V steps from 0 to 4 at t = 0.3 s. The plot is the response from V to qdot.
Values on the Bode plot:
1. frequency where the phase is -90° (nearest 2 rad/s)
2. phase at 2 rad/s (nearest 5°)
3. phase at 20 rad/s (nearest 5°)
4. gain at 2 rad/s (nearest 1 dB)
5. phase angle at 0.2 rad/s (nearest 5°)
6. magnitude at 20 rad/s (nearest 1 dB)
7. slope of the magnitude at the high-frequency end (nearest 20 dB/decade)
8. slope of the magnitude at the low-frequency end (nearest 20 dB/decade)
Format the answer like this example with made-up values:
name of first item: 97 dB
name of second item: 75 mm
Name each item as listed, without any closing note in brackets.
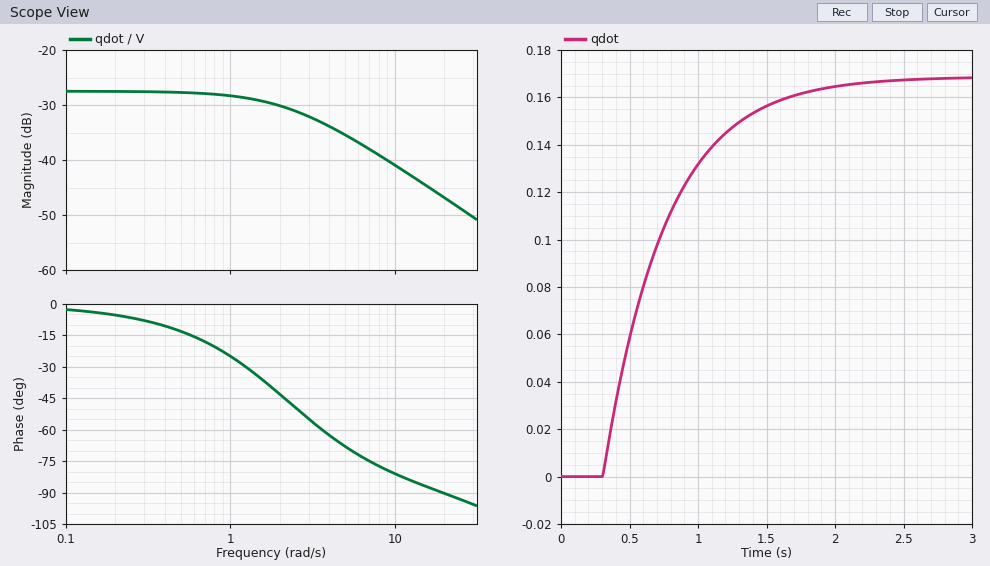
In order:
frequency where the phase is -90°: 20 rad/s
phase at 2 rad/s: -45°
phase at 20 rad/s: -90°
gain at 2 rad/s: -30 dB
phase angle at 0.2 rad/s: -5°
magnitude at 20 rad/s: -47 dB
slope of the magnitude at the high-frequency end: -20 dB/decade
slope of the magnitude at the low-frequency end: 0 dB/decade
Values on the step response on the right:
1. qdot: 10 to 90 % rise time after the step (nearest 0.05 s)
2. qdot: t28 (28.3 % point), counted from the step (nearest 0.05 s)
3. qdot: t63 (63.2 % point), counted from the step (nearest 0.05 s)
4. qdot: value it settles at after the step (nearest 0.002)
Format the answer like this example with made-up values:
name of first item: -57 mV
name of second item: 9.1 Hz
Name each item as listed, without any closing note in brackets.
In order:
qdot: 10 to 90 % rise time after the step: 1.00 s
qdot: t28 (28.3 % point), counted from the step: 0.15 s
qdot: t63 (63.2 % point), counted from the step: 0.45 s
qdot: value it settles at after the step: 0.168
